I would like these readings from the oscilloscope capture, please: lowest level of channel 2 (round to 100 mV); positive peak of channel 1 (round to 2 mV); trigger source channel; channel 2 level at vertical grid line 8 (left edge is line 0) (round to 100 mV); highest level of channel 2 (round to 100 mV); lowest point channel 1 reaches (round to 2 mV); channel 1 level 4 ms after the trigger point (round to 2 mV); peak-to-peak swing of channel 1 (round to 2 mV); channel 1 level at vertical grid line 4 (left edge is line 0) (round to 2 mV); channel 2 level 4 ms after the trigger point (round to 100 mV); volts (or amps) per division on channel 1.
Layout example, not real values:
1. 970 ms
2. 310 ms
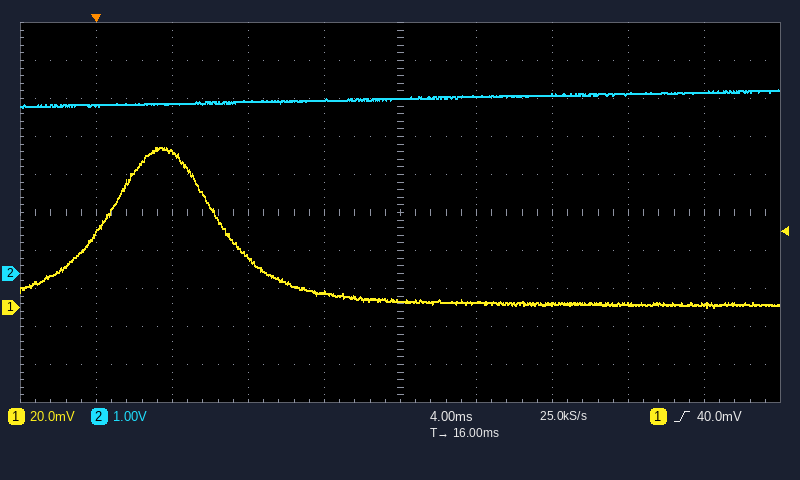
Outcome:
1. 4.4 V
2. 84 mV
3. channel 1
4. 4.7 V
5. 4.8 V
6. 0 mV
7. 82 mV
8. 84 mV
9. 8 mV
10. 4.5 V
11. 20 mV
